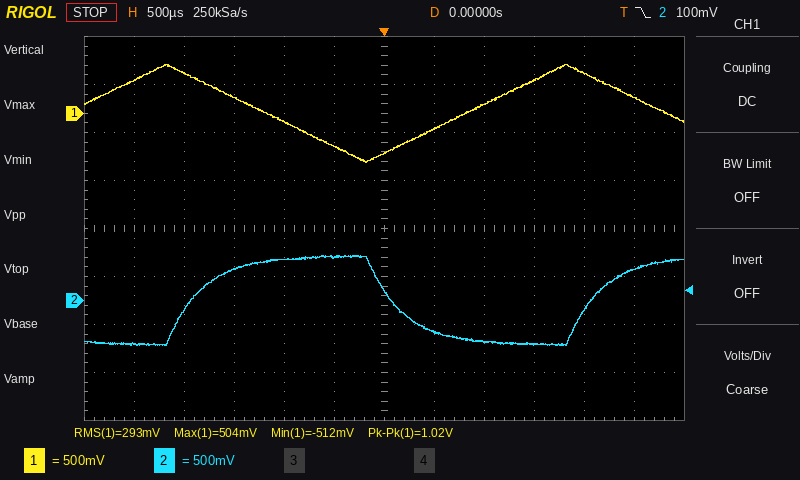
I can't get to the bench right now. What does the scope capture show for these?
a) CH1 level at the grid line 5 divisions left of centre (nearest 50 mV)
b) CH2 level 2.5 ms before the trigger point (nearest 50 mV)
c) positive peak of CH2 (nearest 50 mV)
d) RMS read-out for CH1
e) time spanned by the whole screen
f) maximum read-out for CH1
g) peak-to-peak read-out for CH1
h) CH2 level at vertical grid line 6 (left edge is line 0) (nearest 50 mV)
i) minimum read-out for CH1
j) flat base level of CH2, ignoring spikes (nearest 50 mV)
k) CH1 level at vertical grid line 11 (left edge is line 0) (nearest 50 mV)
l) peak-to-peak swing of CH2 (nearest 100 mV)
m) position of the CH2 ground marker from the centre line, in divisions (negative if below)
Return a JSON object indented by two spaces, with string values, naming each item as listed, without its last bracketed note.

{
  "CH1 level at the grid line 5 divisions left of centre": "350 mV",
  "CH2 level 2.5 ms before the trigger point": "-450 mV",
  "positive peak of CH2": "450 mV",
  "RMS read-out for CH1": "293 mV",
  "time spanned by the whole screen": "6 ms",
  "maximum read-out for CH1": "504 mV",
  "peak-to-peak read-out for CH1": "1.02 V",
  "CH2 level at vertical grid line 6 (left edge is line 0)": "100 mV",
  "minimum read-out for CH1": "-512 mV",
  "flat base level of CH2, ignoring spikes": "-450 mV",
  "CH1 level at vertical grid line 11 (left edge is line 0)": "150 mV",
  "peak-to-peak swing of CH2": "900 mV",
  "position of the CH2 ground marker from the centre line, in divisions": "-1.5 div"
}
